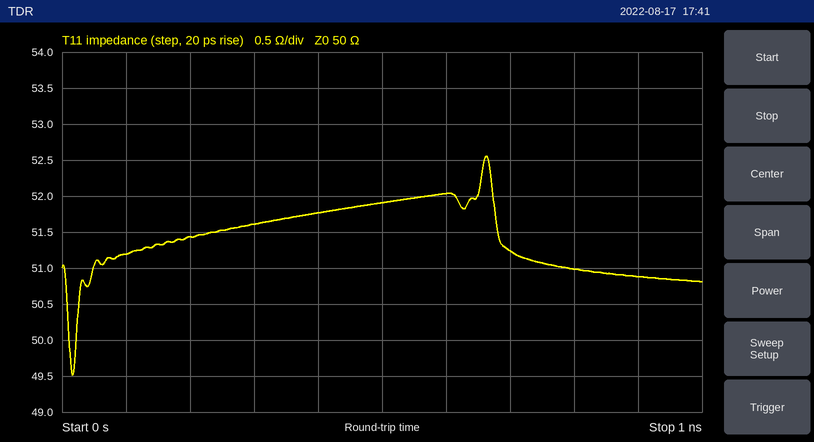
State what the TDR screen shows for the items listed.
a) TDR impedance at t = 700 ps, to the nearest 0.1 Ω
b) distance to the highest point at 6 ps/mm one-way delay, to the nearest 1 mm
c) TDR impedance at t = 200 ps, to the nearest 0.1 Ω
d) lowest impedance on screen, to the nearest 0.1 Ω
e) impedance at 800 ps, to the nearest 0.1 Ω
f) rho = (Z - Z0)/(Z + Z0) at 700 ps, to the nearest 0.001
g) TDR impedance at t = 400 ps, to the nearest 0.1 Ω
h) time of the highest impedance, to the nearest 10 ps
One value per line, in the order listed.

51.2 Ω
55 mm
51.4 Ω
49.5 Ω
51.0 Ω
+0.012
51.8 Ω
660 ps
